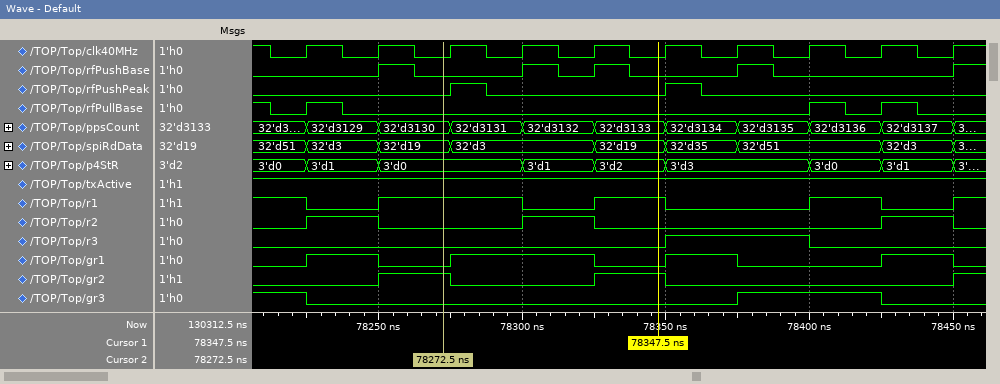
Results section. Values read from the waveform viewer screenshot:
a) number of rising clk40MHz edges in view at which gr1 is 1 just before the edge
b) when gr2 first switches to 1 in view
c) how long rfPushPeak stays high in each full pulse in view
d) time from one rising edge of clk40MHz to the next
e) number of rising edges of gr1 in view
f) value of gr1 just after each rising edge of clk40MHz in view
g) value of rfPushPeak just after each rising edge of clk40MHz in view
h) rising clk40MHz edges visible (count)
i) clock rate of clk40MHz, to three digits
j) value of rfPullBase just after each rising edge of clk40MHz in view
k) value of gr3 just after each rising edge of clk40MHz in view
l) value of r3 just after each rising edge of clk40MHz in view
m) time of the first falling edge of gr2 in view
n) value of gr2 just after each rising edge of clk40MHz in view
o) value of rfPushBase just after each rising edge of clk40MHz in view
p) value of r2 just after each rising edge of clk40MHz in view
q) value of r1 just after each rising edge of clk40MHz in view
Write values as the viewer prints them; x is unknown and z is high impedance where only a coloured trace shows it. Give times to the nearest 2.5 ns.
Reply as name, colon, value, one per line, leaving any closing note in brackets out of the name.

number of rising clk40MHz edges in view at which gr1 is 1 just before the edge: 5
when gr2 first switches to 1 in view: 78250 ns
how long rfPushPeak stays high in each full pulse in view: 12.5 ns, 12.5 ns
time from one rising edge of clk40MHz to the next: 25 ns
number of rising edges of gr1 in view: 4
value of gr1 just after each rising edge of clk40MHz in view: 1 0 1 1 0 1 0 0 1 0
value of rfPushPeak just after each rising edge of clk40MHz in view: 0 0 1 0 0 1 0 0 0 0
rising clk40MHz edges visible: 10
clock rate of clk40MHz, to three digits: 40.0 MHz
value of rfPullBase just after each rising edge of clk40MHz in view: 1 0 0 0 0 0 0 1 1 0
value of gr3 just after each rising edge of clk40MHz in view: 0 0 0 0 0 0 1 1 0 0
value of r3 just after each rising edge of clk40MHz in view: 0 0 0 0 0 1 1 0 0 0
time of the first falling edge of gr2 in view: 78275 ns
value of gr2 just after each rising edge of clk40MHz in view: 0 1 0 0 1 0 0 0 0 1
value of rfPushBase just after each rising edge of clk40MHz in view: 0 1 0 1 1 0 1 0 0 1
value of r2 just after each rising edge of clk40MHz in view: 1 0 0 1 0 0 0 0 1 0
value of r1 just after each rising edge of clk40MHz in view: 0 1 1 0 1 0 0 1 0 1
